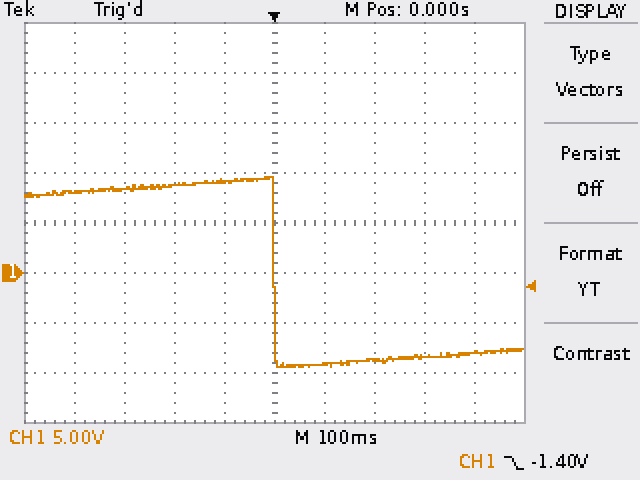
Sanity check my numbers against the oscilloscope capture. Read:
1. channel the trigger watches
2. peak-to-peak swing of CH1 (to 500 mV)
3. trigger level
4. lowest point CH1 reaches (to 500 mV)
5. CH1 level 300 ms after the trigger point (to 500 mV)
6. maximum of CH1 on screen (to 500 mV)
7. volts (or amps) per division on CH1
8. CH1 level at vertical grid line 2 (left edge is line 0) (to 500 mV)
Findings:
CH1
19.0 V
-1.40 V
-9.5 V
-8.5 V
9.5 V
5 V
8.5 V
